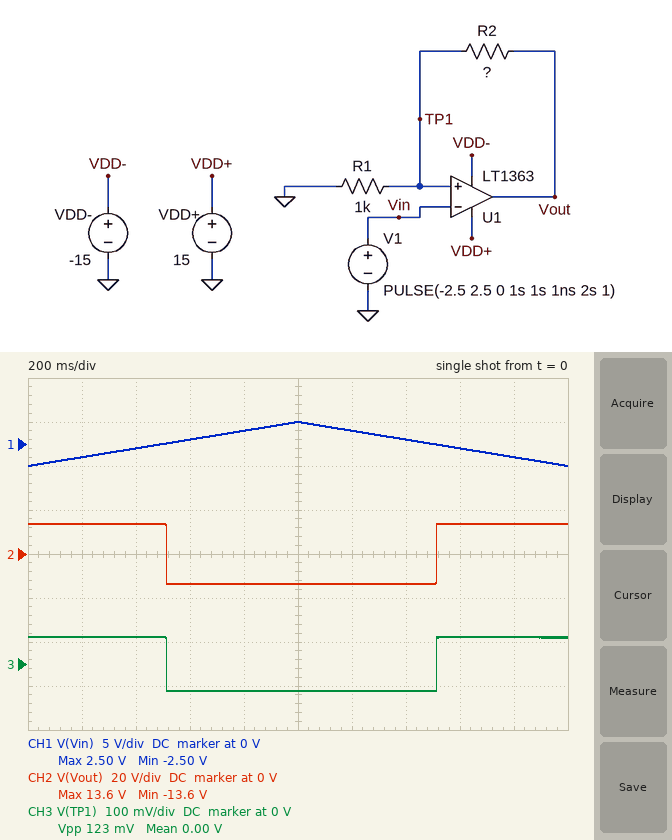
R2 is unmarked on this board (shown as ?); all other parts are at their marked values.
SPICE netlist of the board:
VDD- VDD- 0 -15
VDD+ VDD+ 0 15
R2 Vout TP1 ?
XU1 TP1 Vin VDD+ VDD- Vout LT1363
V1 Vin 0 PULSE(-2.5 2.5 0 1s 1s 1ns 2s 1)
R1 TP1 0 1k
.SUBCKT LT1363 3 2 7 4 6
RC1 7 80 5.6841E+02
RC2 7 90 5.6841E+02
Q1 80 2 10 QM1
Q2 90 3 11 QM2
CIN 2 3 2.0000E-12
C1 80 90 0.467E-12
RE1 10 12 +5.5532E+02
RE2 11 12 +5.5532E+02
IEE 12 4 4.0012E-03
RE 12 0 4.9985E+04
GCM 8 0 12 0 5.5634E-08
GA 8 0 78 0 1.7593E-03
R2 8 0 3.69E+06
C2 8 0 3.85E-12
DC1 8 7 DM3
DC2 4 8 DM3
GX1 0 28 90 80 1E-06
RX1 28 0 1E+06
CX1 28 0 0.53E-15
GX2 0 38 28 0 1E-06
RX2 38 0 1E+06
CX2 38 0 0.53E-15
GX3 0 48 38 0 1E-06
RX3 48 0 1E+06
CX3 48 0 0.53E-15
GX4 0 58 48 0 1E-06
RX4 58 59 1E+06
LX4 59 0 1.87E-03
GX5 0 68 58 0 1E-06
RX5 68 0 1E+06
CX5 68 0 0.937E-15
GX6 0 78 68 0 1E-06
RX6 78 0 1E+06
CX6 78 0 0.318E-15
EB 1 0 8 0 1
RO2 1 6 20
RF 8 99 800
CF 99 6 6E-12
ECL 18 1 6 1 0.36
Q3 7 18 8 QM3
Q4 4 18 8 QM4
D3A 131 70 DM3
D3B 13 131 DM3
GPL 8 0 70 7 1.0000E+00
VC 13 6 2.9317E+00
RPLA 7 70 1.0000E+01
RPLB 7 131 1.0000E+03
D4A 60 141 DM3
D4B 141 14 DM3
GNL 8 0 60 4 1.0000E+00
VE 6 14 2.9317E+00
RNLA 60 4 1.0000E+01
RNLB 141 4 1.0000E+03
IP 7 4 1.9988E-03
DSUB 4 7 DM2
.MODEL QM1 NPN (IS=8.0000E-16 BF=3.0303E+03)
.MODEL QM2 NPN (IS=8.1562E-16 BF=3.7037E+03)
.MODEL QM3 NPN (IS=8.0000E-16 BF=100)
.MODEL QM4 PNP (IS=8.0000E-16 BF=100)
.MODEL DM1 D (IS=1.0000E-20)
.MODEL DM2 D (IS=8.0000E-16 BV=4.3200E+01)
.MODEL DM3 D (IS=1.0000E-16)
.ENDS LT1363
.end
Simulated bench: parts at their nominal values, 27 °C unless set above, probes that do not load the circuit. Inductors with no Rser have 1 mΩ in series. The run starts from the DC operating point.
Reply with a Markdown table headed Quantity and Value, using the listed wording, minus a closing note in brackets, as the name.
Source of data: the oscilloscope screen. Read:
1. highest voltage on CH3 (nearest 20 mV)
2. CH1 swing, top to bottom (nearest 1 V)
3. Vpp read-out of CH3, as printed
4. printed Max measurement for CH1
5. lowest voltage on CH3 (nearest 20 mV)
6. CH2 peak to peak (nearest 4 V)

| Quantity | Value |
|---|---|
| highest voltage on CH3 | 60 mV |
| CH1 swing, top to bottom | 5 V |
| Vpp read-out of CH3, as printed | 123 mV |
| printed Max measurement for CH1 | 2.50 V |
| lowest voltage on CH3 | -60 mV |
| CH2 peak to peak | 28 V |
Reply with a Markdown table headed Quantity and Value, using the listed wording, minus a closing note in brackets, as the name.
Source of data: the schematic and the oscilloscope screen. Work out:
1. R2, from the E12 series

| Quantity | Value |
|---|---|
| R2, from the E12 series | 220 kΩ |
